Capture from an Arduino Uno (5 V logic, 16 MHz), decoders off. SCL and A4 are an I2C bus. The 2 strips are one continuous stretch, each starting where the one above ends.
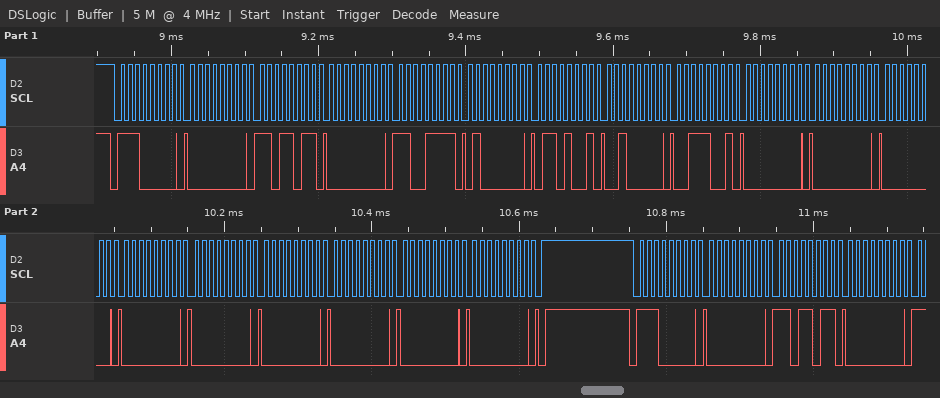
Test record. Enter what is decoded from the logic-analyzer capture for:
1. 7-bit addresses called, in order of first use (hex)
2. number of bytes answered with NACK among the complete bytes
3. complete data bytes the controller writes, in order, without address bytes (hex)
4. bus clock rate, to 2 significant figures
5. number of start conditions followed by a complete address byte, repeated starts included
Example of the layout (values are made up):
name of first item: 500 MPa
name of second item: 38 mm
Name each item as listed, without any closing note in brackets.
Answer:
7-bit addresses called, in order of first use: 0x70
number of bytes answered with NACK among the complete bytes: 0
complete data bytes the controller writes, in order, without address bytes: 00 DB 00 CF 40 69 20 39 00 00 00 00 00 00 00 00 00 00 DB 00
bus clock rate, to 2 significant figures: 100 kHz
number of start conditions followed by a complete address byte, repeated starts included: 2
